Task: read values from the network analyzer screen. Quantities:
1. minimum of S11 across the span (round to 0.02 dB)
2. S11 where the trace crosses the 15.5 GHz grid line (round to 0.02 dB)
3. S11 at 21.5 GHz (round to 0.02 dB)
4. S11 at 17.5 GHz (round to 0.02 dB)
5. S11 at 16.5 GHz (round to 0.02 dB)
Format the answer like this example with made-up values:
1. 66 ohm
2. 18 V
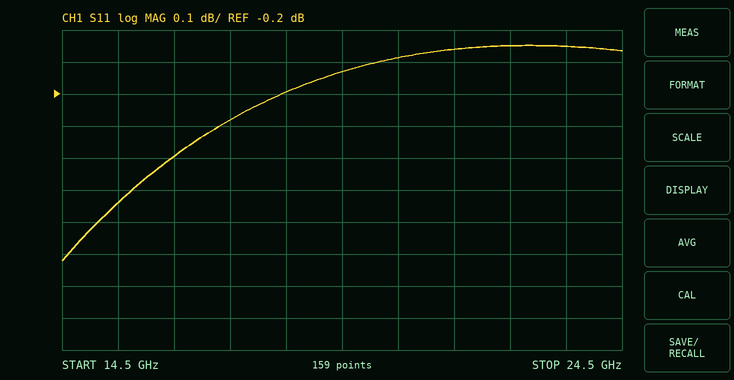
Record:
1. -0.72 dB
2. -0.54 dB
3. -0.06 dB
4. -0.28 dB
5. -0.40 dB
